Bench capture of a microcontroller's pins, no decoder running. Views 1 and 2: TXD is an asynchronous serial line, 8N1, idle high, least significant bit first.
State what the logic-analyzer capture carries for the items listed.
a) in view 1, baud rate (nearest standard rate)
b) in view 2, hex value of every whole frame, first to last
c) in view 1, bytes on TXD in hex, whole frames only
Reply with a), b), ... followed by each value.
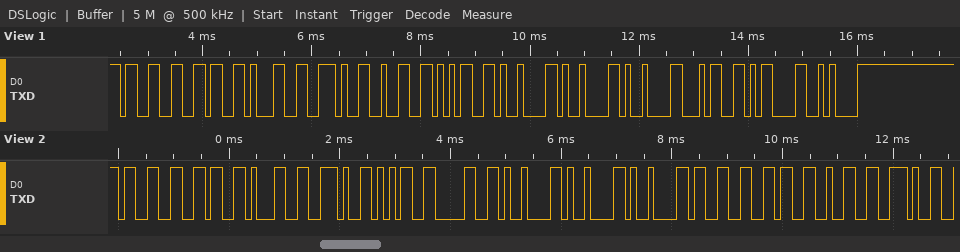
a) 9600 baud
b) 33 36 31 2E 35 30 09 09 09 33 36 32 2E
c) 33 36 31 2E 32 35 09 09 09 34 0D 0A
